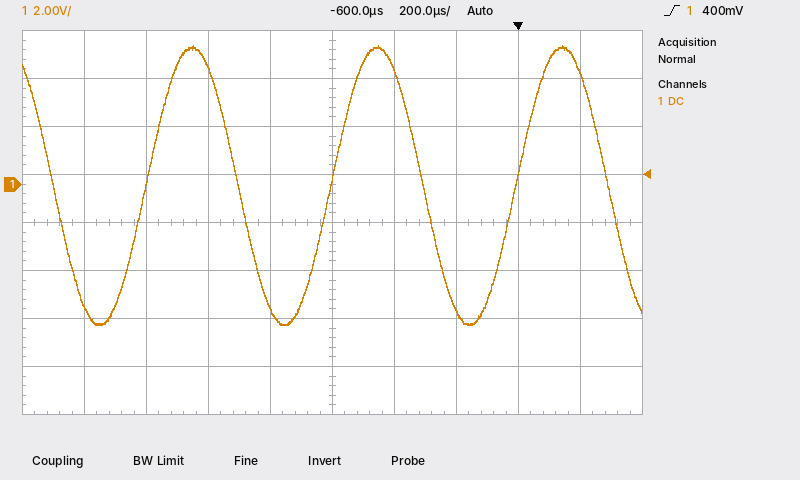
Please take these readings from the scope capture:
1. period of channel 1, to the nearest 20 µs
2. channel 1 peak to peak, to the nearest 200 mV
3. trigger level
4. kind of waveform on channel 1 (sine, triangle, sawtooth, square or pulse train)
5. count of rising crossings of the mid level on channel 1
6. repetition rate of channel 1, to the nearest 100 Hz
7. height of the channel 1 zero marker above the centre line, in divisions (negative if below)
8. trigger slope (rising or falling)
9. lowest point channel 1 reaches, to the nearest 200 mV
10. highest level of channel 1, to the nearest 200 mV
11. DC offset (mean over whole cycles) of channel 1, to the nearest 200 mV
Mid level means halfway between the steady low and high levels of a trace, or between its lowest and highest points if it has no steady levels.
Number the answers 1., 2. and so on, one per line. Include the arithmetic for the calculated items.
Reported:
1. 600 µs
2. 5.8 V − (-5.8 V) = 11.6 V
3. 400 mV
4. sine
5. 3
6. 1 / 600 µs ≈ 1.7 kHz
7. +0.8 div
8. rising
9. -5.8 V
10. 5.8 V
11. (5.8 V + (-5.8 V)) / 2 ≈ 0.0 V
